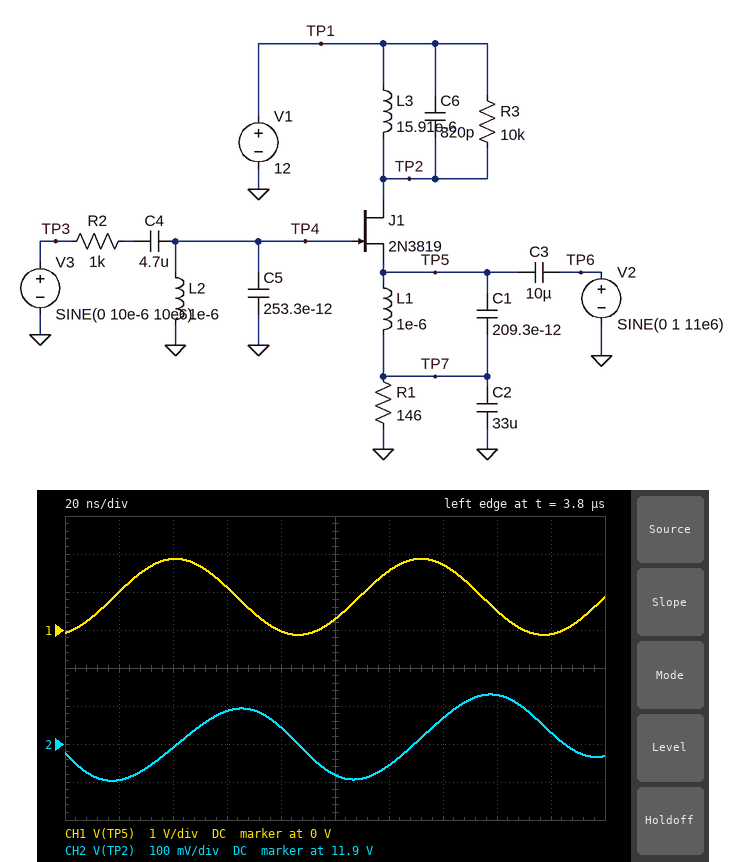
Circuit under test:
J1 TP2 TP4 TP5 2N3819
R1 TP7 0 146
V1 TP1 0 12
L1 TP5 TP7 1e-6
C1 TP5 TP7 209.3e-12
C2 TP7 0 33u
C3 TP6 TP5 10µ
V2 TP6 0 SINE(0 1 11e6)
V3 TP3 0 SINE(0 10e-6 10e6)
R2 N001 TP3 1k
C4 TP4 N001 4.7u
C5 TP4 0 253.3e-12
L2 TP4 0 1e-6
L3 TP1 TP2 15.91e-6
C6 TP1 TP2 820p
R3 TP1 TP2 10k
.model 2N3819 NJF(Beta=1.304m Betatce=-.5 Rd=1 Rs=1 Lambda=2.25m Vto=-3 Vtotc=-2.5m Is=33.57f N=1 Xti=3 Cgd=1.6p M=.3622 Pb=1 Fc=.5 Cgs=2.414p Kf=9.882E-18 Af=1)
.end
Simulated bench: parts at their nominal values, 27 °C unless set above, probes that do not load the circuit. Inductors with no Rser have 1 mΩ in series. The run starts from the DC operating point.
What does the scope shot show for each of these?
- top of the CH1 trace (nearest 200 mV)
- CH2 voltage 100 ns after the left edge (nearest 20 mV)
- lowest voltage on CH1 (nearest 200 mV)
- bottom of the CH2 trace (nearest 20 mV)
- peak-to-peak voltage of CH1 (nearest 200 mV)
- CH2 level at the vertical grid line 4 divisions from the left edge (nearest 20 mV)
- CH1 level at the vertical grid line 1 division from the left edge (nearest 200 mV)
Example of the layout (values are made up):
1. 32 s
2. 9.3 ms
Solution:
1. 1.8 V
2. 11.82 V
3. -200 mV
4. 11.80 V
5. 2.0 V
6. 11.94 V
7. 1.0 V
